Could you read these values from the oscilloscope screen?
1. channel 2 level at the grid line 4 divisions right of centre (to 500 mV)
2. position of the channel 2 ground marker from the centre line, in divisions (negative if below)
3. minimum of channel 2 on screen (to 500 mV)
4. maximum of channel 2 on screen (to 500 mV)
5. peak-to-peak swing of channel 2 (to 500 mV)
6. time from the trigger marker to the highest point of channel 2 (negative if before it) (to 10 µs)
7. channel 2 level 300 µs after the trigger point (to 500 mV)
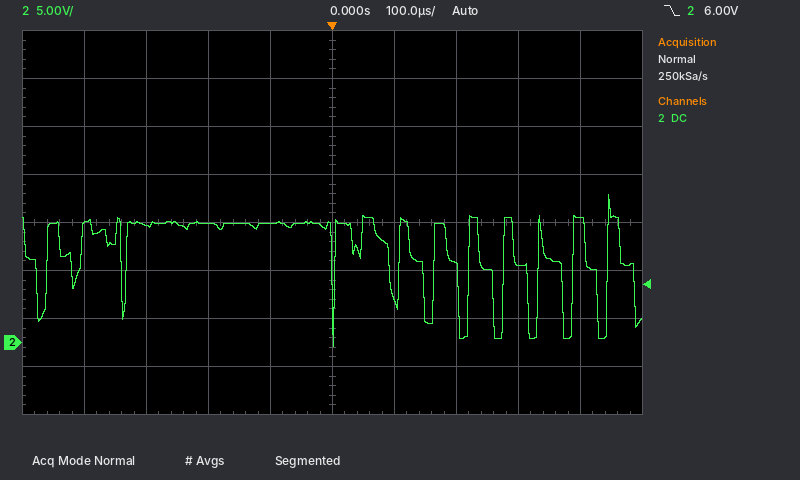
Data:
13.0 V
-2.5 div
-500 mV
15.5 V
16.0 V
+450 µs
8.0 V
